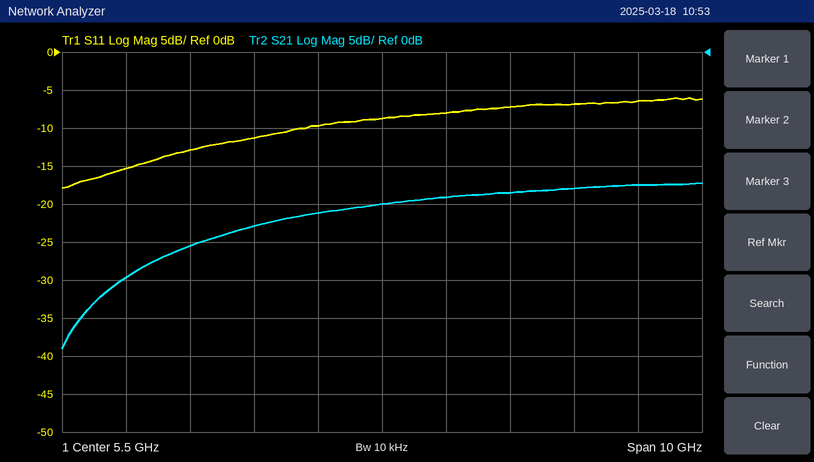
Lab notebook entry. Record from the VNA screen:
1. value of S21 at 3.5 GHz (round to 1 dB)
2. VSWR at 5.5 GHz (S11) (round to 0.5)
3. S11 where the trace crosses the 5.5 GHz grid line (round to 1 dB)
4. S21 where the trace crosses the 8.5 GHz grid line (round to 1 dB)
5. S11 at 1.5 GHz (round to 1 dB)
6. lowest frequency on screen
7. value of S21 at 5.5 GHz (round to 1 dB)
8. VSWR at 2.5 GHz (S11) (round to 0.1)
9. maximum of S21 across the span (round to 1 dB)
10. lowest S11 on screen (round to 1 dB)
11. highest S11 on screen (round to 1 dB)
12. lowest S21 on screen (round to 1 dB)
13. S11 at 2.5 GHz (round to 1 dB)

-23 dB
2.0
-9 dB
-18 dB
-15 dB
500 MHz
-20 dB
1.6
-17 dB
-18 dB
-6 dB
-39 dB
-13 dB
